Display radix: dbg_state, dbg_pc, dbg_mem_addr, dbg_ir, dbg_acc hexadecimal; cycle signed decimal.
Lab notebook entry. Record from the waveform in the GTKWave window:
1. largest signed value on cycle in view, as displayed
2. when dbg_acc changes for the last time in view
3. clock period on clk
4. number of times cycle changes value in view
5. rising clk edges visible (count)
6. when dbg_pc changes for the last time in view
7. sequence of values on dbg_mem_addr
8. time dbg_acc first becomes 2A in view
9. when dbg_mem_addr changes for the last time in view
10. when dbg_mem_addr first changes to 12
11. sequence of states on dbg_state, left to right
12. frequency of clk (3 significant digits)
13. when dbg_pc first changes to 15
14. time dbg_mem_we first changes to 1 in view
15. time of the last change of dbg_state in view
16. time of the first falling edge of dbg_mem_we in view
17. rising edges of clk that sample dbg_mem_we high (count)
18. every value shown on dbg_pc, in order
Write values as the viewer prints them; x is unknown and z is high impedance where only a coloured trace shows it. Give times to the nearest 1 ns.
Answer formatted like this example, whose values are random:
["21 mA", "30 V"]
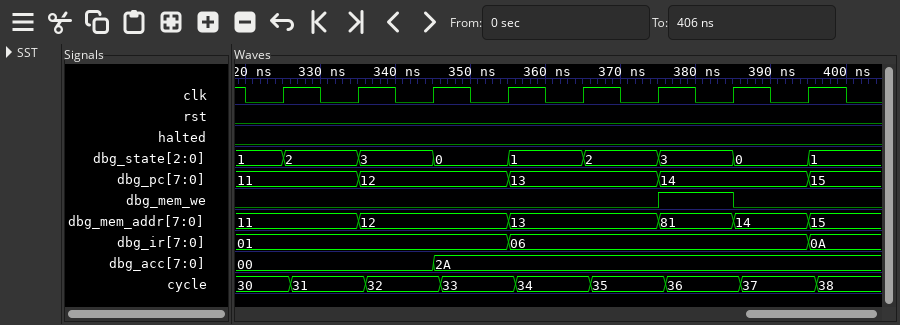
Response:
["38", "345 ns", "10 ns", "8", "8", "395 ns", "11, 12, 13, 81, 14, 15", "345 ns", "395 ns", "335 ns", "1, 2, 3, 0, 1, 2, 3, 0, 1", "100 MHz", "395 ns", "375 ns", "395 ns", "385 ns", "1", "11, 12, 13, 14, 15"]
